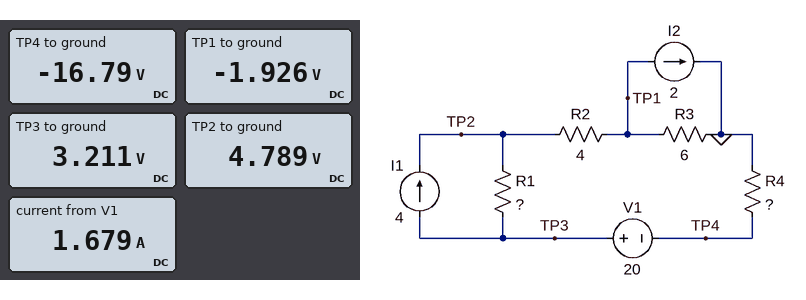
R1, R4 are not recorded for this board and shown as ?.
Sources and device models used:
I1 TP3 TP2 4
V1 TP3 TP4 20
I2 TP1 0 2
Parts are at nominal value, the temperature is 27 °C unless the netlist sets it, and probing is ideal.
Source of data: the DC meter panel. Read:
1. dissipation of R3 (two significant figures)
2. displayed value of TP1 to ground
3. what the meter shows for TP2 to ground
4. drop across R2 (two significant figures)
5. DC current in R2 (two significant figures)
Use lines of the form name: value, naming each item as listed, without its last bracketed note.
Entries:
dissipation of R3: 620 mW
displayed value of TP1 to ground: -1.926 V
what the meter shows for TP2 to ground: 4.789 V
drop across R2: 6.7 V
DC current in R2: 1.7 A
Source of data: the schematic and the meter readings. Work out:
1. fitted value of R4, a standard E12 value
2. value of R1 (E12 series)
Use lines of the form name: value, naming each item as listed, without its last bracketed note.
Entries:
fitted value of R4, a standard E12 value: 10 Ω
value of R1: 0.68 Ω
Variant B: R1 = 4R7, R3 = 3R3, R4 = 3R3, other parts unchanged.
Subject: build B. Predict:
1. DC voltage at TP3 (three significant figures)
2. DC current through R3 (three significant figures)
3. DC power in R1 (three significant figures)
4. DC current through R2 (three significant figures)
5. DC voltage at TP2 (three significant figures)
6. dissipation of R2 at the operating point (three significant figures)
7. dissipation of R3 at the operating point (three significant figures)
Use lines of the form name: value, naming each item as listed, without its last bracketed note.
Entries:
DC voltage at TP3: 10.2 V
DC current through R3: 967 mA
DC power in R1: 5.01 W
DC current through R2: 2.97 A
DC voltage at TP2: 15.1 V
dissipation of R2 at the operating point: 35.2 W
dissipation of R3 at the operating point: 3.09 W
